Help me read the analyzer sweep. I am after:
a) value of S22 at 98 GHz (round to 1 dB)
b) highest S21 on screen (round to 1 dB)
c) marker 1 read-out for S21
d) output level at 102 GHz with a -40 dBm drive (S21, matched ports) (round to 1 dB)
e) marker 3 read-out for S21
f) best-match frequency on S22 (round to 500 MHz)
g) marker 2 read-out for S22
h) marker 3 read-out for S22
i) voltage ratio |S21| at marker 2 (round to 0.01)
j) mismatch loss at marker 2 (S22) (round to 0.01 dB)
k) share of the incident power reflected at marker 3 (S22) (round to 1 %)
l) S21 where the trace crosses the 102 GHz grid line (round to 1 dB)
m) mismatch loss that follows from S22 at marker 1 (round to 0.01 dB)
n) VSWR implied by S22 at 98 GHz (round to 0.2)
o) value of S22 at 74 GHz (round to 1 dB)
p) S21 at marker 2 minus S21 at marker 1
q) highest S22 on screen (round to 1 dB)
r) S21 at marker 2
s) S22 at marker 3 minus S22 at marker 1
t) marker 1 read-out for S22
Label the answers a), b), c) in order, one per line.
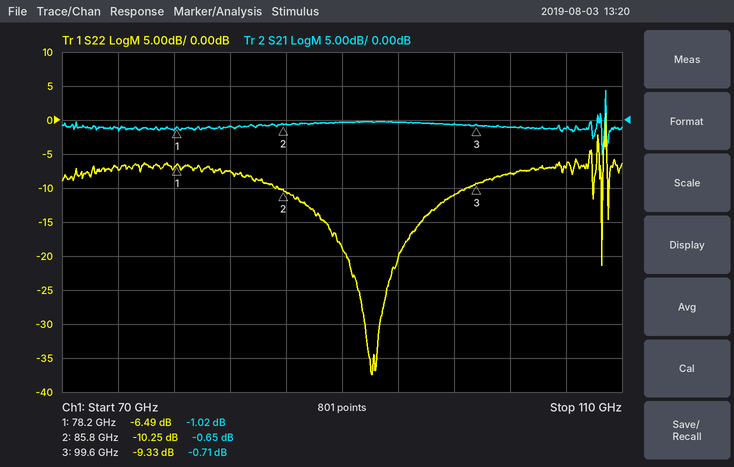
a) -11 dB
b) 4 dB
c) -1.02 dB
d) -41 dBm
e) -0.71 dB
f) 92.0 GHz
g) -10.25 dB
h) -9.33 dB
i) 0.93
j) 0.43 dB
k) 12 %
l) -1 dB
m) 1.10 dB
n) 1.8
o) -7 dB
p) 0.37 dB
q) 1 dB
r) -0.65 dB
s) -2.84 dB
t) -6.49 dB
